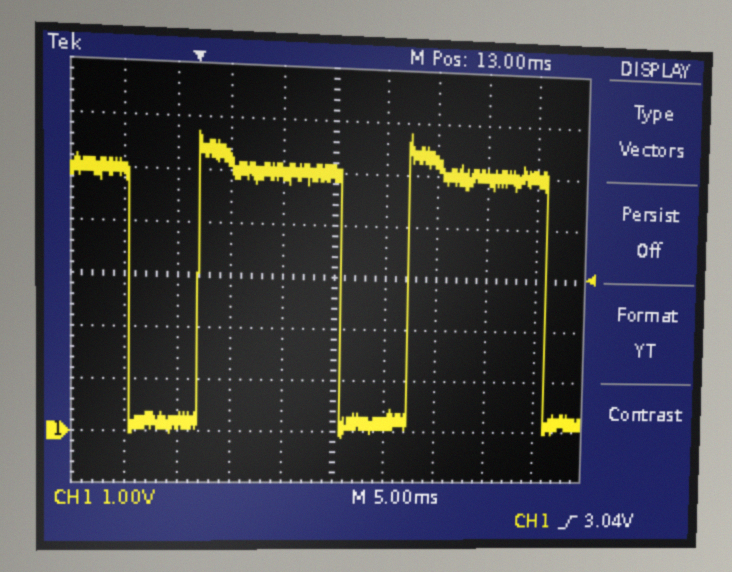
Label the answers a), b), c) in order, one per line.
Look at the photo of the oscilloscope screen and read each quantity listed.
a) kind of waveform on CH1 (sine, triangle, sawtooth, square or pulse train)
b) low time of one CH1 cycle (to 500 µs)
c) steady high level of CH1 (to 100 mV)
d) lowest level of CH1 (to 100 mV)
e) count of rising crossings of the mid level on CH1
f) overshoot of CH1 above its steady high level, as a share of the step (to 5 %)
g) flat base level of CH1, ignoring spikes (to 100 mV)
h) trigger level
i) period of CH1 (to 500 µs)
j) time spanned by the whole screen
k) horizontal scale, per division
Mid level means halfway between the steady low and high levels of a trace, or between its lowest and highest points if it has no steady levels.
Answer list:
a) pulse train
b) 6.5 ms
c) 5.0 V
d) -100 mV
e) 2
f) 15 %
g) 200 mV
h) 3.04 V
i) 20.5 ms
j) 50 ms
k) 5 ms
